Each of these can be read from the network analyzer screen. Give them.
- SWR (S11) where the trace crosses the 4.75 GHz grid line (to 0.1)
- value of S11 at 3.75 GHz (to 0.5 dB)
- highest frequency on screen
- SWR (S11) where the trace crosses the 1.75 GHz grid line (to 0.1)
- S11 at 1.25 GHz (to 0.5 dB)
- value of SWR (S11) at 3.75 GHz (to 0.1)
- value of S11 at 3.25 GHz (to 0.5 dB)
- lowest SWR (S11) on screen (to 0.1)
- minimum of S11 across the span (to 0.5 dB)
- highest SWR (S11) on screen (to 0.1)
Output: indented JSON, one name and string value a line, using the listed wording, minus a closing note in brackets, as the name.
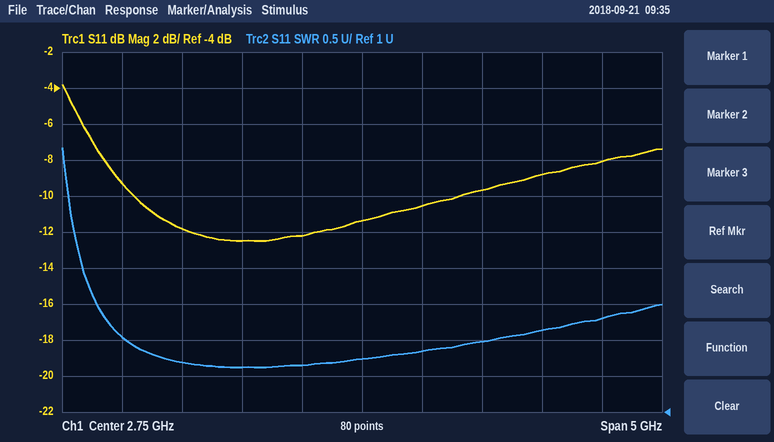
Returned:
{
  "SWR (S11) where the trace crosses the 4.75 GHz grid line": "2.3",
  "value of S11 at 3.75 GHz": "-9.5 dB",
  "highest frequency on screen": "5.25 GHz",
  "SWR (S11) where the trace crosses the 1.75 GHz grid line": "1.6",
  "S11 at 1.25 GHz": "-12.0 dB",
  "value of SWR (S11) at 3.75 GHz": "2.0",
  "value of S11 at 3.25 GHz": "-10.5 dB",
  "lowest SWR (S11) on screen": "1.6",
  "minimum of S11 across the span": "-12.5 dB",
  "highest SWR (S11) on screen": "4.7"
}
